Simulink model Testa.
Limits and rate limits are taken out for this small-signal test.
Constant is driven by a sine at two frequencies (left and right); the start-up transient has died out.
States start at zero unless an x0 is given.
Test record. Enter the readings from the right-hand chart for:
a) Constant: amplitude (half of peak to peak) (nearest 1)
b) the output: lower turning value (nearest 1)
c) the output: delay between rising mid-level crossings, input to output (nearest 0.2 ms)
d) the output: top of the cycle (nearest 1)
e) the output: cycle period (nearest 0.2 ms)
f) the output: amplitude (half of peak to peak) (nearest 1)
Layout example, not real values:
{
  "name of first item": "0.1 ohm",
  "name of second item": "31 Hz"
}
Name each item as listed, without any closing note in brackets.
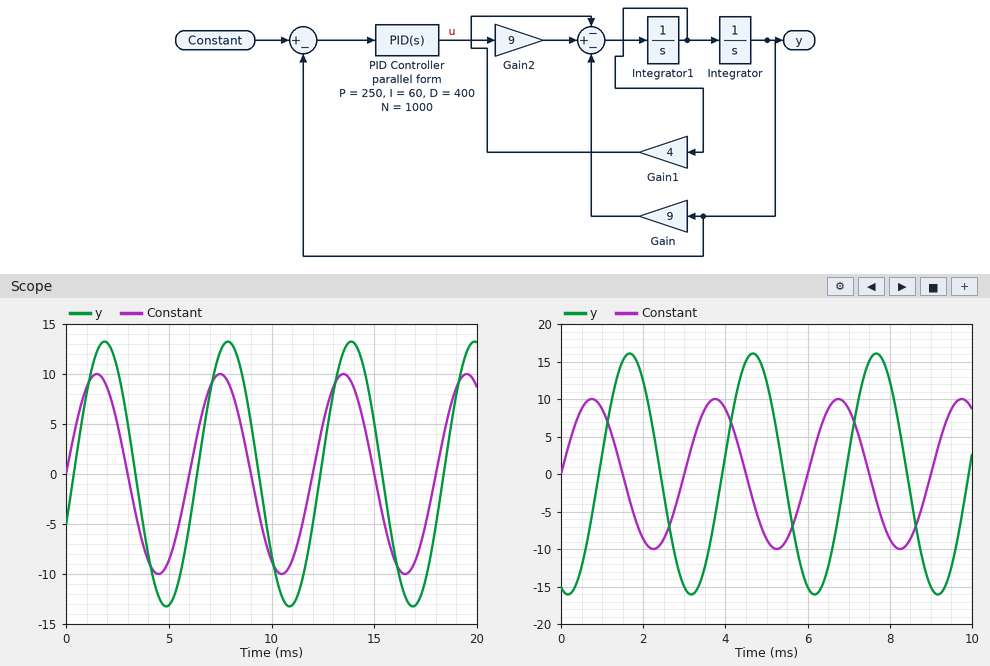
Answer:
{
  "Constant: amplitude (half of peak to peak)": "10",
  "the output: lower turning value": "-16",
  "the output: delay between rising mid-level crossings, input to output": "1.0 ms",
  "the output: top of the cycle": "16",
  "the output: cycle period": "3.0 ms",
  "the output: amplitude (half of peak to peak)": "16"
}
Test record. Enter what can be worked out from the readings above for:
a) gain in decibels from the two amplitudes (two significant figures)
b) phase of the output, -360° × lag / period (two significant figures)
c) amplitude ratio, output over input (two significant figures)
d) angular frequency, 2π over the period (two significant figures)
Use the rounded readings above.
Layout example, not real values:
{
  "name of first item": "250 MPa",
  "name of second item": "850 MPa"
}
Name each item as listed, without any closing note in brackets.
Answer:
{
  "gain in decibels from the two amplitudes": "4.1 dB",
  "phase of the output, -360° × lag / period": "-120°",
  "amplitude ratio, output over input": "1.6",
  "angular frequency, 2π over the period": "2.1 rad/ms"
}
